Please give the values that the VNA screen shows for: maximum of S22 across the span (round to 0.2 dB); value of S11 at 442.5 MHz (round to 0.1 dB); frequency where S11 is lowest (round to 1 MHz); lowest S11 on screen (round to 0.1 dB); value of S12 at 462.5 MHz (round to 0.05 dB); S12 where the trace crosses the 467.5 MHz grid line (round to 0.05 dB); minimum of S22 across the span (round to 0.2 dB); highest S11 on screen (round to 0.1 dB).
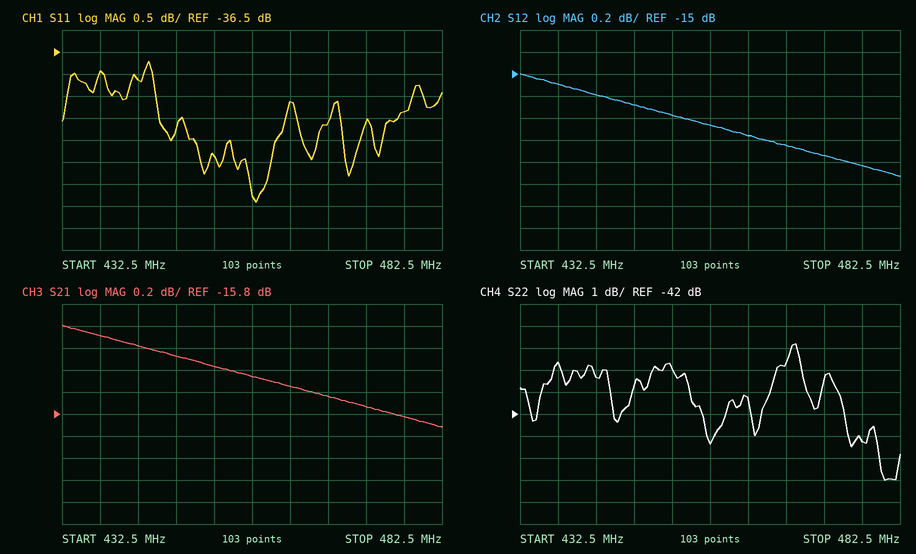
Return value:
-38.8 dB
-37.1 dB
458 MHz
-39.9 dB
-15.55 dB
-15.65 dB
-45.0 dB
-36.7 dB
